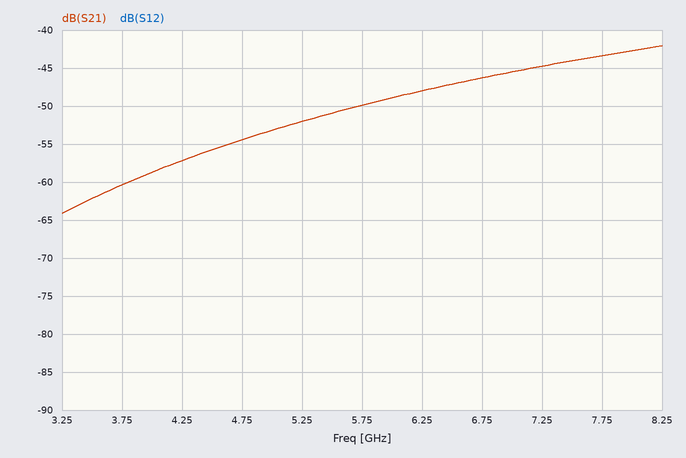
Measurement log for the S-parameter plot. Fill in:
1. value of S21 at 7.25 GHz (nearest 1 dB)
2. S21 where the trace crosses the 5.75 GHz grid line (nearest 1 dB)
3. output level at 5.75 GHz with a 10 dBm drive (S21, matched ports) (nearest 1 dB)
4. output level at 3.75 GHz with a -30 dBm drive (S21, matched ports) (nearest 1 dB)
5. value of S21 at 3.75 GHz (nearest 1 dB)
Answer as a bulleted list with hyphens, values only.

- -45 dB
- -50 dB
- -40 dBm
- -90 dBm
- -60 dB
